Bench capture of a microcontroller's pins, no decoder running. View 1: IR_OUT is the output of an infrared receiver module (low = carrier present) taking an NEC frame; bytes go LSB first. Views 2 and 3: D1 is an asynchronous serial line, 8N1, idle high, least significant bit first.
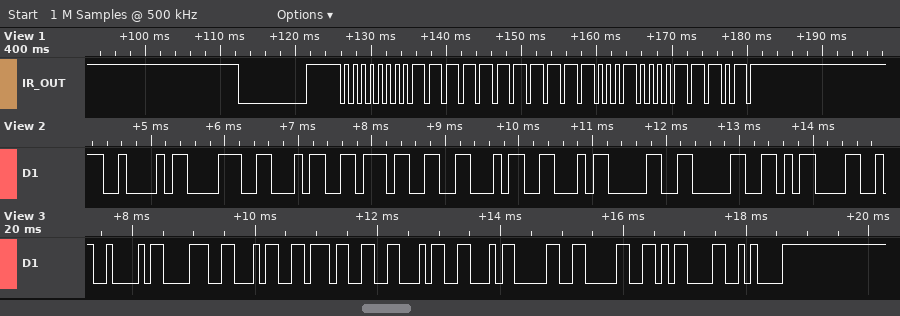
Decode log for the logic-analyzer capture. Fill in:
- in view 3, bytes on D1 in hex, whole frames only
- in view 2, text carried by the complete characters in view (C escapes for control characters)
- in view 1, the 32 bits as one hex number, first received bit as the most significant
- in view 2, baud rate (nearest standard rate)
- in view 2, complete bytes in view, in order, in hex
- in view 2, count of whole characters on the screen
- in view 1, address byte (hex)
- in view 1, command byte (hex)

0x42 0x38 0x34 0x37 0x46 0x46 0x30 0x30 0x0D 0x0A
"B847FF00\r"
0x00FFE21D
9600 baud
42 38 34 37 46 46 30 30 0D
9
0x00
0x47
